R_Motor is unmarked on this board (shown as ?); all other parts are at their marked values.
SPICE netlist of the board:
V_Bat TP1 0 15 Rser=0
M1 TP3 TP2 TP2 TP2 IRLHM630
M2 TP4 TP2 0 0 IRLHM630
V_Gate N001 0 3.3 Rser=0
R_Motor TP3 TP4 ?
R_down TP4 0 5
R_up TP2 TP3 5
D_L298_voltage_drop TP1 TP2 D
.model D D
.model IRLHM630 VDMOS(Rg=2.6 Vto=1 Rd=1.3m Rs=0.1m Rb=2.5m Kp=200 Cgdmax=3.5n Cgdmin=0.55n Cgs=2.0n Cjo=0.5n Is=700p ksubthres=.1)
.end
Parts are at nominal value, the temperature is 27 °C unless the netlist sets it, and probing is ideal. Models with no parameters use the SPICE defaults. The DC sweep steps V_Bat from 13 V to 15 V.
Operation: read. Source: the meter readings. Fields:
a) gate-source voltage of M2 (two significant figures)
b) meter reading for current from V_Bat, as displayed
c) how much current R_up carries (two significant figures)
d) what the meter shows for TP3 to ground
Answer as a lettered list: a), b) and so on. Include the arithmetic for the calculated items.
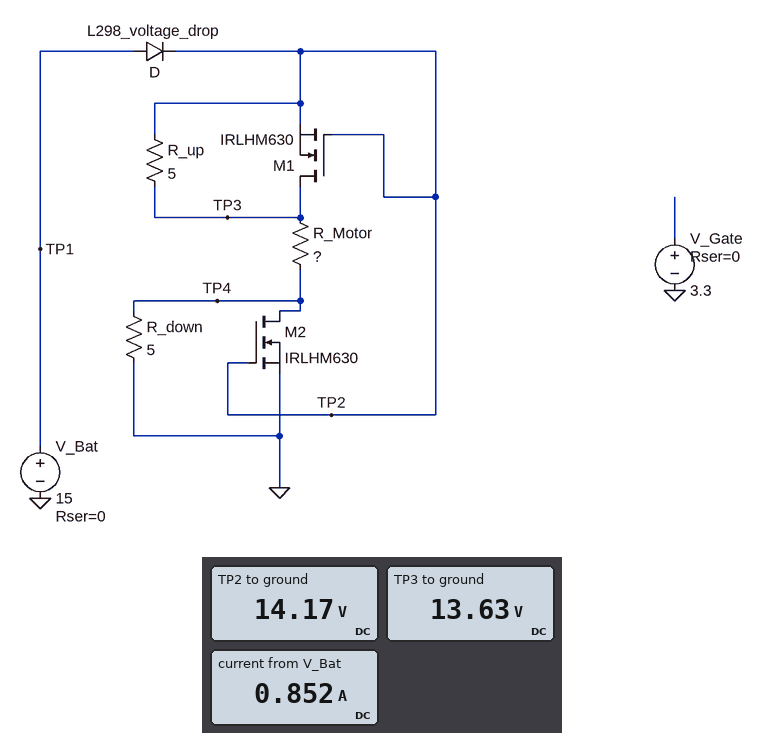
a) 14.17 V = 14 V
b) 0.852 A
c) (14.17 V - 13.63 V) / 5 Ω = 110 mA
d) 13.63 V
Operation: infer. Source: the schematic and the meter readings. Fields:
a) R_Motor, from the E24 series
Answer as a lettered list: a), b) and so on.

a) 16 Ω
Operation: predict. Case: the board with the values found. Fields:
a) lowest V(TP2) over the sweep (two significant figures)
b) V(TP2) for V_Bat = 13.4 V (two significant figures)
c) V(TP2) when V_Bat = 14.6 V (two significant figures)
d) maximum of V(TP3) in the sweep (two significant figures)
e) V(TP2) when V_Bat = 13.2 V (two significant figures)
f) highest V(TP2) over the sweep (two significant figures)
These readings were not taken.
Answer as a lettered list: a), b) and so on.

a) 12 V
b) 13 V
c) 14 V
d) 14 V
e) 12 V
f) 14 V
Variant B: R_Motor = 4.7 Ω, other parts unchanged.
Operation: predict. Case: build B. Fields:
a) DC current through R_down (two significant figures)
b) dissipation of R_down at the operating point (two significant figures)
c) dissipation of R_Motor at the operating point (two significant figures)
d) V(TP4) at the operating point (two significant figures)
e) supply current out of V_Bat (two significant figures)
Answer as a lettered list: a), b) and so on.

a) 1.0 mA
b) 5.3 µW
c) 39 W
d) 5.1 mV
e) 2.9 A
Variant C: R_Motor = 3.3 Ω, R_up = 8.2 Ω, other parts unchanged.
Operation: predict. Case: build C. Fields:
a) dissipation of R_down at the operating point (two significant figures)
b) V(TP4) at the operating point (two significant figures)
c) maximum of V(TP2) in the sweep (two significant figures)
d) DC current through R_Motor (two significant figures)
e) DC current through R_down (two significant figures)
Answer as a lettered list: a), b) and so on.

a) 11 µW
b) 7.3 mV
c) 14 V
d) 4.1 A
e) 1.5 mA
